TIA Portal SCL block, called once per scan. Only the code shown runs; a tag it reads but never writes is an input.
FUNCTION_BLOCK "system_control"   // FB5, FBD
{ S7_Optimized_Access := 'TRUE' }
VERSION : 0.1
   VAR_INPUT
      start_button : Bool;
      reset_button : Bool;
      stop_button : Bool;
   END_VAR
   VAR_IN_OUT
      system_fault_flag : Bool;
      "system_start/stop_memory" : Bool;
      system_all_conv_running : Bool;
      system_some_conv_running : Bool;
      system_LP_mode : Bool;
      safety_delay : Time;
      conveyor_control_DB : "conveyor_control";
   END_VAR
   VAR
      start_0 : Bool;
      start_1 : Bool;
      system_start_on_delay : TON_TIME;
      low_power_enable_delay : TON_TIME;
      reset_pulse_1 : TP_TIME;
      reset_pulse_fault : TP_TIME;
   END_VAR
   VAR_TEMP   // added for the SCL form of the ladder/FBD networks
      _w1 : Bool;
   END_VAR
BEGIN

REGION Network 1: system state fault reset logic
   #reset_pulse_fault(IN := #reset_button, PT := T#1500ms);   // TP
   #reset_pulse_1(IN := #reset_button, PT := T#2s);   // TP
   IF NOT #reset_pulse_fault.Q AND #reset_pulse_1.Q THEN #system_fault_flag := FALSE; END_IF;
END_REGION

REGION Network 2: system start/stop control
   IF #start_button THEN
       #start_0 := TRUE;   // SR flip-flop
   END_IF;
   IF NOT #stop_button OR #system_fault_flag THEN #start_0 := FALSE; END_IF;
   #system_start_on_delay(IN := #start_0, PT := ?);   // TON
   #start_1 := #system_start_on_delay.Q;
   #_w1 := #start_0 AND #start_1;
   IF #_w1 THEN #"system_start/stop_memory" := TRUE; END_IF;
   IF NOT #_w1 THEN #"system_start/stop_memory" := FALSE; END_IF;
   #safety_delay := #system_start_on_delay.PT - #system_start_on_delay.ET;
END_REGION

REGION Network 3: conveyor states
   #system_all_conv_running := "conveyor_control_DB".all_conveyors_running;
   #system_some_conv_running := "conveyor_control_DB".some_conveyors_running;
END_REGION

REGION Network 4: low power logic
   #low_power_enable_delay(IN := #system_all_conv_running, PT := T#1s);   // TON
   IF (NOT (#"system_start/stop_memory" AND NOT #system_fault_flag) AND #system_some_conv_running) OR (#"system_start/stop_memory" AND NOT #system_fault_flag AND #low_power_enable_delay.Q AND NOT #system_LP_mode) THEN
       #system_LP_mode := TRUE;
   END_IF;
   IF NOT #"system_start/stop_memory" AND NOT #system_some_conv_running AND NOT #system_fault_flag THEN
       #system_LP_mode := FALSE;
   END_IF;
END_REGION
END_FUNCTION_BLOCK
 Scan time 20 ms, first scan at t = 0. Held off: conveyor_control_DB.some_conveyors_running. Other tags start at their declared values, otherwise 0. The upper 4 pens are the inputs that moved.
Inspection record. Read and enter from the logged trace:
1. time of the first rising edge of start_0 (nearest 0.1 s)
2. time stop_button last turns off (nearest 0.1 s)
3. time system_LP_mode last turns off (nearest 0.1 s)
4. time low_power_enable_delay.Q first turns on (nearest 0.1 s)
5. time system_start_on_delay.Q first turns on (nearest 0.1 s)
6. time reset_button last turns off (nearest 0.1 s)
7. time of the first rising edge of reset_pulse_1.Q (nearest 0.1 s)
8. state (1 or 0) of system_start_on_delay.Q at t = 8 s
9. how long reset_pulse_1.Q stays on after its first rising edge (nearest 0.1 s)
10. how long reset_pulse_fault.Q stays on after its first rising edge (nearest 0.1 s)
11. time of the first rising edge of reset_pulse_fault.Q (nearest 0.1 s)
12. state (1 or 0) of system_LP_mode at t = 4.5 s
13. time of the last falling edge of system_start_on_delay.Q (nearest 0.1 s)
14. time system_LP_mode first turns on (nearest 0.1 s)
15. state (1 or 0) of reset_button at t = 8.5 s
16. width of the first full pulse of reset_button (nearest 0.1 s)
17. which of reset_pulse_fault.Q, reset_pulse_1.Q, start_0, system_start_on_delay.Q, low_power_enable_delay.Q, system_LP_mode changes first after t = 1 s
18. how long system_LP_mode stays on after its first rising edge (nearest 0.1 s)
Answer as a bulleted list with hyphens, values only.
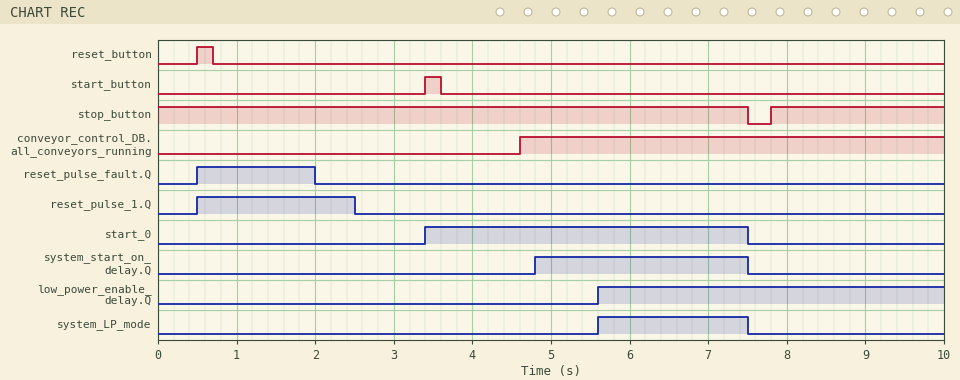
- 3.4 s
- 7.5 s
- 7.5 s
- 5.6 s
- 4.8 s
- 0.7 s
- 0.5 s
- 0
- 2.0 s
- 1.5 s
- 0.5 s
- 0
- 7.5 s
- 5.6 s
- 0
- 0.2 s
- reset_pulse_fault.Q
- 1.9 s
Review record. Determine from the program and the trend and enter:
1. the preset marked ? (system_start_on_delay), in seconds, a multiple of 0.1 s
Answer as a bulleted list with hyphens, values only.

- 1.4 s
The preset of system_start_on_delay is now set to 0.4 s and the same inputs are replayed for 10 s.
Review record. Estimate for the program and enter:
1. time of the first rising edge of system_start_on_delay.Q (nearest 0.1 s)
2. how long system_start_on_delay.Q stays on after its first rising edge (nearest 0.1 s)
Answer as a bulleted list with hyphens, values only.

- 3.8 s
- 3.7 s
